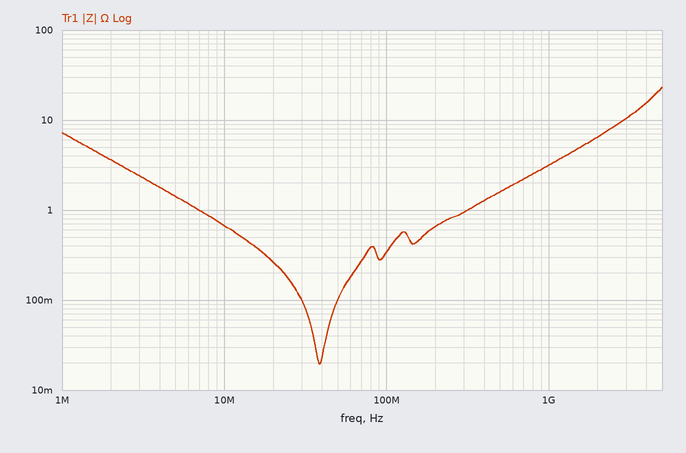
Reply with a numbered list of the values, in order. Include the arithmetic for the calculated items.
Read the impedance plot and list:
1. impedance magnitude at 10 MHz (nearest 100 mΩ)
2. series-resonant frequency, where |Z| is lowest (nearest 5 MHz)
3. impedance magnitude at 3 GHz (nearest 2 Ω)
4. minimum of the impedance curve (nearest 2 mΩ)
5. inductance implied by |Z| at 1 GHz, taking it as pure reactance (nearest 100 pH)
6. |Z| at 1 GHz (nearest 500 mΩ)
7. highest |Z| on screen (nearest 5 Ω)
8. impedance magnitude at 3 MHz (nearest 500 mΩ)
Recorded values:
1. 700 mΩ
2. 40 MHz
3. 10 Ω
4. 20 mΩ
5. L = 3.0 Ω/(2π × 1 GHz) ≈ 477 pH, so 500 pH to the nearest 100 pH
6. 3.0 Ω
7. 25 Ω
8. 2.5 Ω
